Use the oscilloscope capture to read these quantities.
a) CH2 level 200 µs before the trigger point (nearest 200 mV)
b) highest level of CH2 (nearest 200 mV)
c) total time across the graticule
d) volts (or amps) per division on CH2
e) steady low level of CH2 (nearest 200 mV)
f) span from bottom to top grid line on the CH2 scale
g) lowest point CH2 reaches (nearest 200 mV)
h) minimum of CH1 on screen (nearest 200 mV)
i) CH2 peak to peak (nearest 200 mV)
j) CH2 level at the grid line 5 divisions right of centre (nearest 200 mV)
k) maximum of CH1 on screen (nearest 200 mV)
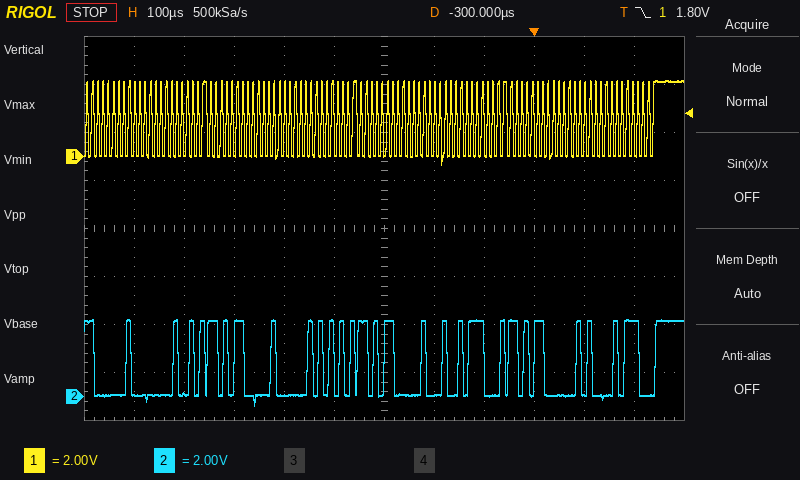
0.0 V
3.2 V
1.2 ms
2 V
0.0 V
16 V
-400 mV
-400 mV
3.6 V
3.2 V
3.2 V
